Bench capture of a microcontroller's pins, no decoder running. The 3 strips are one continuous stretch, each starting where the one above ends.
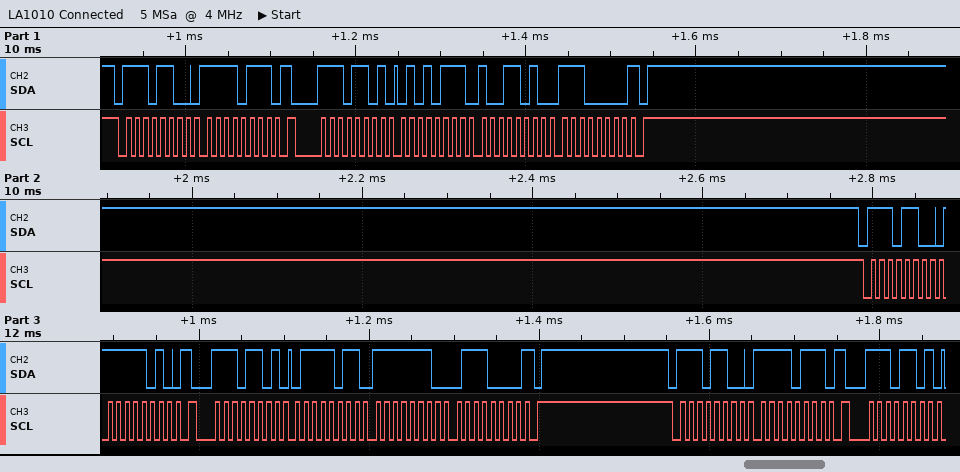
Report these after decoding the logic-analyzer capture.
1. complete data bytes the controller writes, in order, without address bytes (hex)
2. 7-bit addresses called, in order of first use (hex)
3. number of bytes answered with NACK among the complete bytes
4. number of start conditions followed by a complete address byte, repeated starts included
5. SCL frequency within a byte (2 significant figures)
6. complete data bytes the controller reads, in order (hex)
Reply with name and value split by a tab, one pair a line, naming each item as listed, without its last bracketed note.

complete data bytes the controller writes, in order, without address bytes	F7 FA F7
7-bit addresses called, in order of first use	0x76
number of bytes answered with NACK among the complete bytes	2
number of start conditions followed by a complete address byte, repeated starts included	6
SCL frequency within a byte	100 kHz
complete data bytes the controller reads, in order	57 9A E0 7B FE 70
